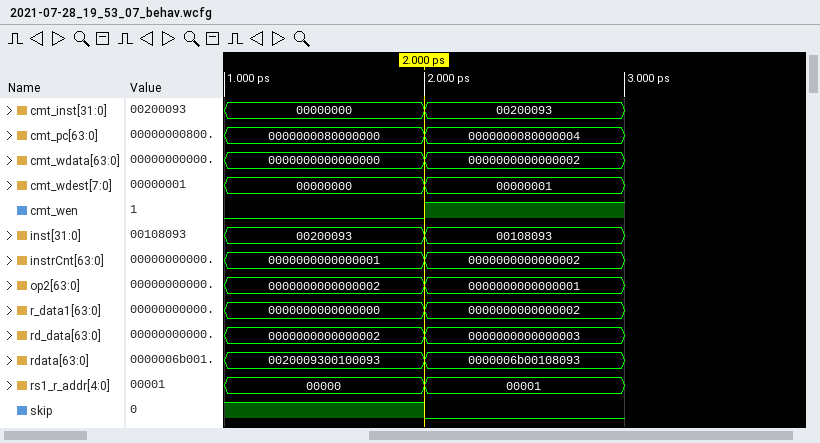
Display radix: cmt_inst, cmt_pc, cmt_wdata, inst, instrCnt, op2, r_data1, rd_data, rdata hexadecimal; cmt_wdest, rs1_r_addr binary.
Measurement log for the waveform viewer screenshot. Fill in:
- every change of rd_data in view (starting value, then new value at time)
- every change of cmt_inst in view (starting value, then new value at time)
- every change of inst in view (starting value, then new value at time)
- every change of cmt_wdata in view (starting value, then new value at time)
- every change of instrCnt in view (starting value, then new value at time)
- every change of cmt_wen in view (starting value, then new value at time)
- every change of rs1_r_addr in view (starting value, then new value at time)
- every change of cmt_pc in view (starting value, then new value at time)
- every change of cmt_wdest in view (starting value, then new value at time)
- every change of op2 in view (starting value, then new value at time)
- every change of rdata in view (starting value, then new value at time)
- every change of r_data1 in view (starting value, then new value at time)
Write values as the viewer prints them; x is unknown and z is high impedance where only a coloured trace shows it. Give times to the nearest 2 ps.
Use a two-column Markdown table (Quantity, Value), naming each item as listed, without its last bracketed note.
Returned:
| Quantity | Value |
|---|---|
| every change of rd_data in view | 0000000000000002, 0000000000000003 at 2 ps |
| every change of cmt_inst in view | 00000000, 00200093 at 2 ps |
| every change of inst in view | 00200093, 00108093 at 2 ps |
| every change of cmt_wdata in view | 0000000000000000, 0000000000000002 at 2 ps |
| every change of instrCnt in view | 0000000000000001, 0000000000000002 at 2 ps |
| every change of cmt_wen in view | 0, 1 at 2 ps |
| every change of rs1_r_addr in view | 00000, 00001 at 2 ps |
| every change of cmt_pc in view | 0000000080000000, 0000000080000004 at 2 ps |
| every change of cmt_wdest in view | 00000000, 00000001 at 2 ps |
| every change of op2 in view | 0000000000000002, 0000000000000001 at 2 ps |
| every change of rdata in view | 0020009300100093, 0000006b00108093 at 2 ps |
| every change of r_data1 in view | 0000000000000000, 0000000000000002 at 2 ps |
